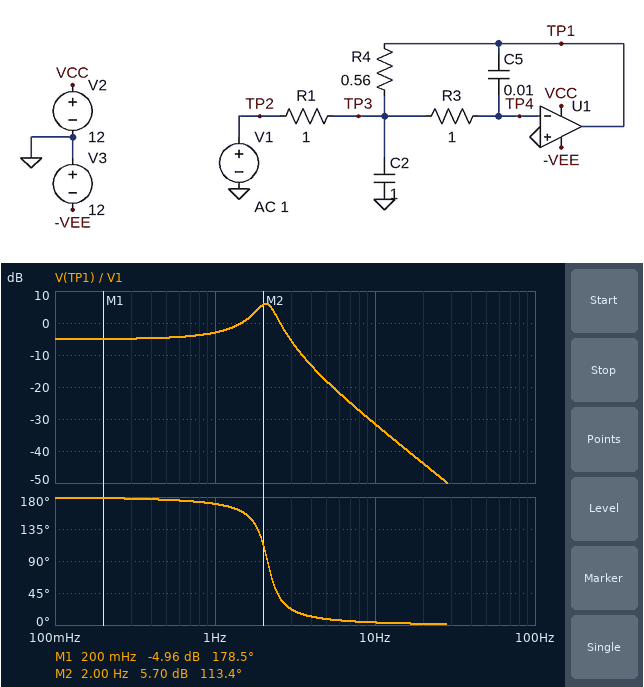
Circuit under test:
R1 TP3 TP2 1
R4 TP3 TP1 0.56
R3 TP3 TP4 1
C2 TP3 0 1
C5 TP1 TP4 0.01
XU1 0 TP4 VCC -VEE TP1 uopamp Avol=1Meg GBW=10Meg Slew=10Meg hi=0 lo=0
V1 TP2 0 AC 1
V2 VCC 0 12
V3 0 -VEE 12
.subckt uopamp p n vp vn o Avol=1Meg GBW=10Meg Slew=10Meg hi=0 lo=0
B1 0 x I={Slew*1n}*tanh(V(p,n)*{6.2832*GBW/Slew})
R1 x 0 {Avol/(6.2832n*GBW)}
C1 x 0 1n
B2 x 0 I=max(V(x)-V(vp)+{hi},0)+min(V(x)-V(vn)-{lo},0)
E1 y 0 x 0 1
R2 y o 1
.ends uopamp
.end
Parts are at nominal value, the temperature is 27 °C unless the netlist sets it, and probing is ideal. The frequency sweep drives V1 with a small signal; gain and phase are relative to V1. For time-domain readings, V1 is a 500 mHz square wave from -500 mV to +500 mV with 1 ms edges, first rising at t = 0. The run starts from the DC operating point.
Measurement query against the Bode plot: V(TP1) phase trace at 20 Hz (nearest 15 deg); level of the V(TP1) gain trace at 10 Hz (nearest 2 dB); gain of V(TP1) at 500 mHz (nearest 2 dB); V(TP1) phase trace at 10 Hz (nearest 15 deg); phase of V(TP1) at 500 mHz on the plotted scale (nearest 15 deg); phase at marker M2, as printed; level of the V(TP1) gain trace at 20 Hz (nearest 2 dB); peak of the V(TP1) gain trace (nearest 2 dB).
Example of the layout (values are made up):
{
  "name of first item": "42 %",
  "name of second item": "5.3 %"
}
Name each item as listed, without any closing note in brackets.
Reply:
{
  "V(TP1) phase trace at 20 Hz": "0 deg",
  "level of the V(TP1) gain trace at 10 Hz": "-32 dB",
  "gain of V(TP1) at 500 mHz": "-4 dB",
  "V(TP1) phase trace at 10 Hz": "0 deg",
  "phase of V(TP1) at 500 mHz on the plotted scale": "180 deg",
  "phase at marker M2, as printed": "113.4 deg",
  "level of the V(TP1) gain trace at 20 Hz": "-44 dB",
  "peak of the V(TP1) gain trace": "6 dB"
}
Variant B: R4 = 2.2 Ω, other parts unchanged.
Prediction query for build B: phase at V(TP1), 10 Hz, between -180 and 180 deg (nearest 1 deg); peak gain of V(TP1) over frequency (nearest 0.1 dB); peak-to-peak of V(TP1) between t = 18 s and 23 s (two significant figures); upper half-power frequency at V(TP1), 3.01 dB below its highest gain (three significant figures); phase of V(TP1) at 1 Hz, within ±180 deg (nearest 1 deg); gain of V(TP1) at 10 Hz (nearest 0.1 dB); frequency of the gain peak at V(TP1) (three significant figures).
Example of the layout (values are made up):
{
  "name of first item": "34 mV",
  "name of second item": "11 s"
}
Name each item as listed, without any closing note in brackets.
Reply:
{
  "phase at V(TP1), 10 Hz, between -180 and 180 deg": "2 deg",
  "peak gain of V(TP1) over frequency": "15.8 dB",
  "peak-to-peak of V(TP1) between t = 18 s and 23 s": "4.1 V",
  "upper half-power frequency at V(TP1), 3.01 dB below its highest gain": "1.22 Hz",
  "phase of V(TP1) at 1 Hz, within ±180 deg": "111 deg",
  "gain of V(TP1) at 10 Hz": "-31.8 dB",
  "frequency of the gain peak at V(TP1)": "1.04 Hz"
}
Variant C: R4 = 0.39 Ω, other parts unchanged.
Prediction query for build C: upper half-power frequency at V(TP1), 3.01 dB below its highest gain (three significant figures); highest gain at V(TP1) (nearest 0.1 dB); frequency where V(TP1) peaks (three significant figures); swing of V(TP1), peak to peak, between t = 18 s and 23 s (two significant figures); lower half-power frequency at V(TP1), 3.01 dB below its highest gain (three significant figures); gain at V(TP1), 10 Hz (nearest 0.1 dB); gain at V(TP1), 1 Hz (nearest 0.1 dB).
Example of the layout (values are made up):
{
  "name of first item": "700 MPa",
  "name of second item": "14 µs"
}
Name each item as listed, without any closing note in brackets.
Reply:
{
  "upper half-power frequency at V(TP1), 3.01 dB below its highest gain": "2.84 Hz",
  "highest gain at V(TP1)": "2.8 dB",
  "frequency where V(TP1) peaks": "2.50 Hz",
  "swing of V(TP1), peak to peak, between t = 18 s and 23 s": "940 mV",
  "lower half-power frequency at V(TP1), 3.01 dB below its highest gain": "2.10 Hz",
  "gain at V(TP1), 10 Hz": "-31.4 dB",
  "gain at V(TP1), 1 Hz": "-6.8 dB"
}
